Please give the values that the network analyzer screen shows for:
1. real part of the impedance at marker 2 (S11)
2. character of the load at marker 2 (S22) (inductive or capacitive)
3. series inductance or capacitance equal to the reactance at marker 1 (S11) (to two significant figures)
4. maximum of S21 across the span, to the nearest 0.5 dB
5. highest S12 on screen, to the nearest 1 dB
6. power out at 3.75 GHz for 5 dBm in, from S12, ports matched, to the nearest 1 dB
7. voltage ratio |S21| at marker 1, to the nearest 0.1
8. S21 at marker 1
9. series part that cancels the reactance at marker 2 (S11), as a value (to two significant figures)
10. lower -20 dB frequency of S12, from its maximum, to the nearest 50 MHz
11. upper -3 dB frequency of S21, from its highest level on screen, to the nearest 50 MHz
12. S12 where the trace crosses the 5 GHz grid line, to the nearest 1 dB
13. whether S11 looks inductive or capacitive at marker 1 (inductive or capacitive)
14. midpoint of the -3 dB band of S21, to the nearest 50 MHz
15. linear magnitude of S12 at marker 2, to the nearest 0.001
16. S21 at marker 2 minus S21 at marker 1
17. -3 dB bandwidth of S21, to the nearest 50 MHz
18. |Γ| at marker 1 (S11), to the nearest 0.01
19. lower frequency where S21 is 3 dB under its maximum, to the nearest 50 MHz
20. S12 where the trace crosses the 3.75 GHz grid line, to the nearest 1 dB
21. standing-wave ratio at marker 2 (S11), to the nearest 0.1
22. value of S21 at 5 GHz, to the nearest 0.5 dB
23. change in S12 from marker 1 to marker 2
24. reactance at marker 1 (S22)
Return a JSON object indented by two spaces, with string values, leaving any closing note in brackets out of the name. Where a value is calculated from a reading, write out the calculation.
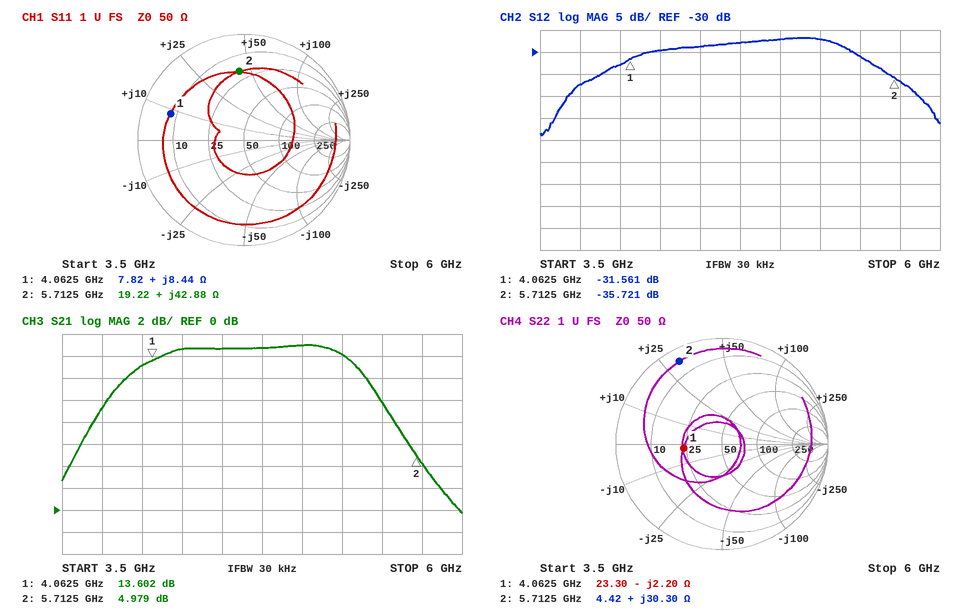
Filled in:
{
  "real part of the impedance at marker 2": "19.22 Ω",
  "character of the load at marker 2 (S22)": "inductive",
  "series inductance or capacitance equal to the reactance at marker 1 (S11)": "L = 8.44 Ω/(2π × 4.0625 GHz) ≈ 331 pH, so 330 pH to two significant figures",
  "maximum of S21 across the span, to the nearest 0.5 dB": "15.0 dB",
  "highest S12 on screen, to the nearest 1 dB": "-27 dB",
  "power out at 3.75 GHz for 5 dBm in, from S12, ports matched, to the nearest 1 dB": "5 dBm + (-37 dB) = -32 dBm",
  "voltage ratio |S21| at marker 1, to the nearest 0.1": "10^(13.602/20) ≈ 4.8",
  "S21 at marker 1": "13.602 dB",
  "series part that cancels the reactance at marker 2 (S11), as a value": "C = 1/(2π × 5.7125 GHz × 42.88 Ω) ≈ 650 fF",
  "lower -20 dB frequency of S12, from its maximum, to the nearest 50 MHz": "3.55 GHz",
  "upper -3 dB frequency of S21, from its highest level on screen, to the nearest 50 MHz": "5.40 GHz",
  "S12 where the trace crosses the 5 GHz grid line, to the nearest 1 dB": "-27 dB",
  "whether S11 looks inductive or capacitive at marker 1": "inductive",
  "midpoint of the -3 dB band of S21, to the nearest 50 MHz": "4.65 GHz",
  "linear magnitude of S12 at marker 2, to the nearest 0.001": "10^(-35.721/20) ≈ 0.016",
  "S21 at marker 2 minus S21 at marker 1": "4.979 − (13.602) = -8.623 dB",
  "-3 dB bandwidth of S21, to the nearest 50 MHz": "5.40 GHz − 3.90 GHz = 1.50 GHz",
  "|Γ| at marker 1 (S11), to the nearest 0.01": "0.74",
  "lower frequency where S21 is 3 dB under its maximum, to the nearest 50 MHz": "3.90 GHz",
  "S12 where the trace crosses the 3.75 GHz grid line, to the nearest 1 dB": "-37 dB",
  "standing-wave ratio at marker 2 (S11), to the nearest 0.1": "4.7",
  "value of S21 at 5 GHz, to the nearest 0.5 dB": "15.0 dB",
  "change in S12 from marker 1 to marker 2": "-35.721 − (-31.561) = -4.160 dB",
  "reactance at marker 1": "-2.20 Ω"
}
